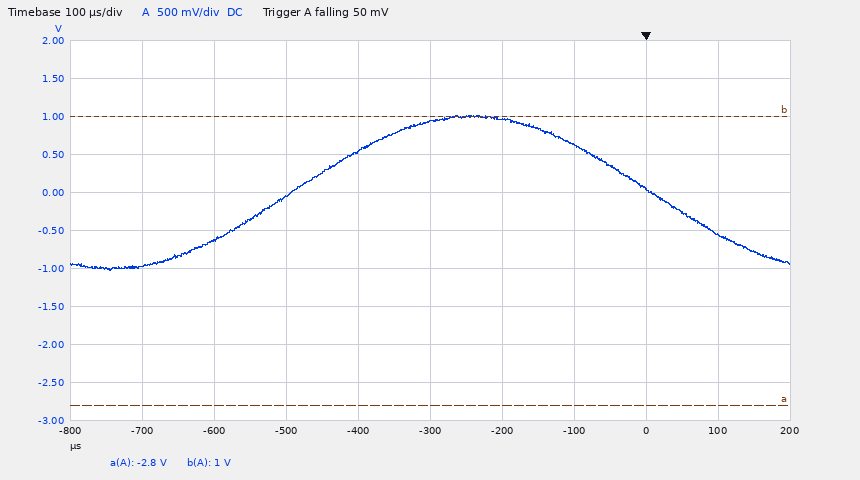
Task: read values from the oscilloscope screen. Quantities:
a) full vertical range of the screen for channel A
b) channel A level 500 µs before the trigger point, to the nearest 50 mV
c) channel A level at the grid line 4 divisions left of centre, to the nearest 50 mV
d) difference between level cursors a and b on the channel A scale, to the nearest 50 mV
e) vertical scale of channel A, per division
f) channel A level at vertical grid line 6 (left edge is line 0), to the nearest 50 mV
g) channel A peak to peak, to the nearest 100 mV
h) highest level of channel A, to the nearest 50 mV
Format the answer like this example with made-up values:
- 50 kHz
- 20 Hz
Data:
- 5 V
- -50 mV
- -950 mV
- 3.80 V
- 500 mV
- 950 mV
- 2.00 V
- 1.00 V
